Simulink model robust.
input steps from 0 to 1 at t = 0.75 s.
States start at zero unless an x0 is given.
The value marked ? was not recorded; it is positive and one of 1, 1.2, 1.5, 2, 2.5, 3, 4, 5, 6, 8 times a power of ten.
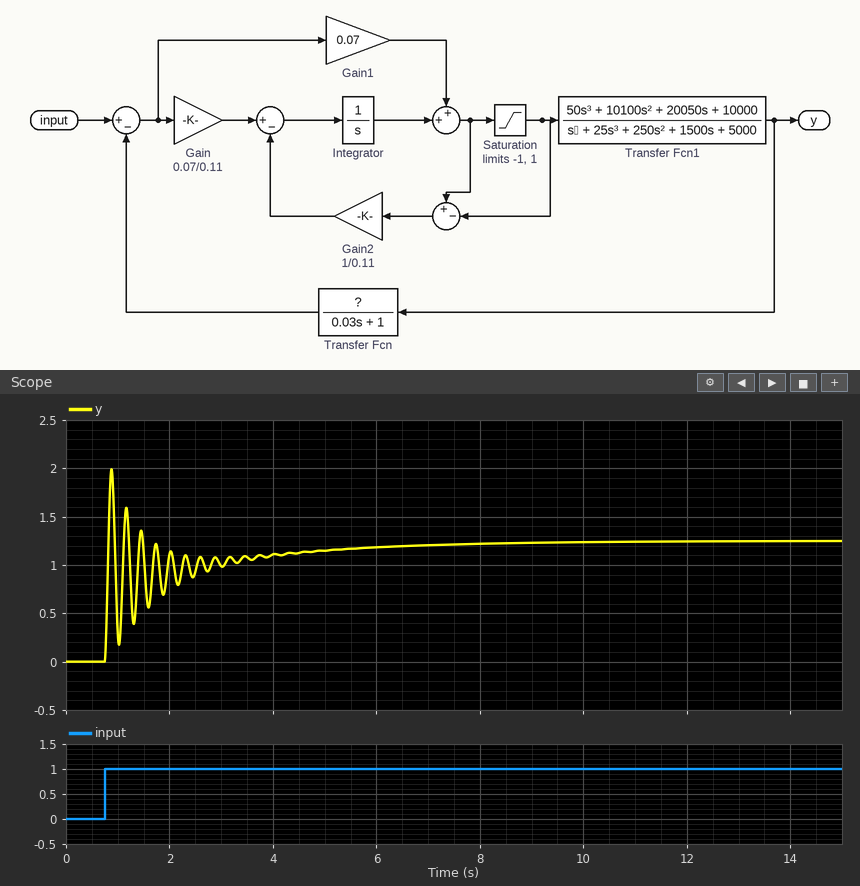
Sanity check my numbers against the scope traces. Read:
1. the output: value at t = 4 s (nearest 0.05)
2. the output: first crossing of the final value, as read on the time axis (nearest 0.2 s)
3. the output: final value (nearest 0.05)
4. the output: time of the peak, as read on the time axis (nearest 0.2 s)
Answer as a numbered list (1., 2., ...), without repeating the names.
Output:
1. 1.10
2. 0.8 s
3. 1.25
4. 0.8 s
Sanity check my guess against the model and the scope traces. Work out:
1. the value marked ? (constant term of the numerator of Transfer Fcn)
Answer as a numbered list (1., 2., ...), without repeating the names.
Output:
1. 0.8
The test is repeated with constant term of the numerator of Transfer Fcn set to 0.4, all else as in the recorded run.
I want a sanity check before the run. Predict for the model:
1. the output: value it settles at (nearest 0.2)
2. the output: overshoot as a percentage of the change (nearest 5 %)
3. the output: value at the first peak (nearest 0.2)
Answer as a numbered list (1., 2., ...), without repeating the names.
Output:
1. 2.0
2. 45 %
3. 2.8
